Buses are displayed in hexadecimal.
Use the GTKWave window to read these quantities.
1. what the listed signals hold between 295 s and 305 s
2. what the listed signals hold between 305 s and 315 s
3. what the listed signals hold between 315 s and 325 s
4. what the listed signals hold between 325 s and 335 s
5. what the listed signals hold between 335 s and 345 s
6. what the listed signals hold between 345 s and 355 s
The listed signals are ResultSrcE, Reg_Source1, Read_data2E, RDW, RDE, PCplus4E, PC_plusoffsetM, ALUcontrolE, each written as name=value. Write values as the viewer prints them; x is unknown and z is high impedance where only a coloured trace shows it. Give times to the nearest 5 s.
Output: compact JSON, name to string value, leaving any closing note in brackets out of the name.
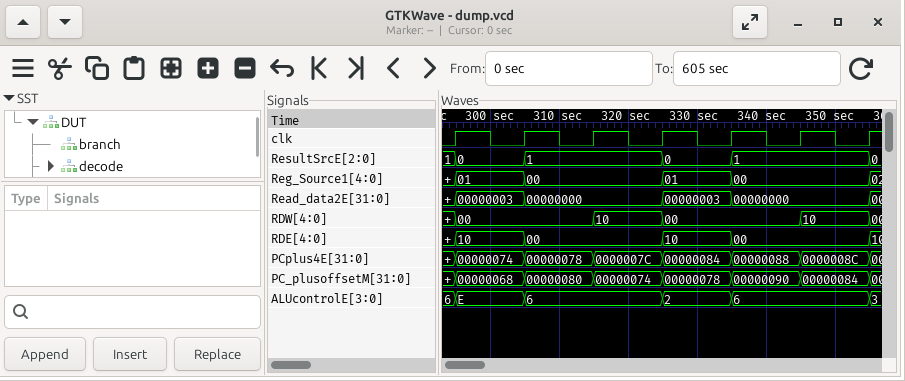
{"what the listed signals hold between 295 s and 305 s": "ResultSrcE=0, Reg_Source1=01, Read_data2E=00000003, RDW=00, RDE=10, PCplus4E=00000074, PC_plusoffsetM=00000068, ALUcontrolE=E", "what the listed signals hold between 305 s and 315 s": "ResultSrcE=1, Reg_Source1=00, Read_data2E=00000000, RDW=00, RDE=00, PCplus4E=00000078, PC_plusoffsetM=00000080, ALUcontrolE=6", "what the listed signals hold between 315 s and 325 s": "ResultSrcE=1, Reg_Source1=00, Read_data2E=00000000, RDW=10, RDE=00, PCplus4E=0000007C, PC_plusoffsetM=00000074, ALUcontrolE=6", "what the listed signals hold between 325 s and 335 s": "ResultSrcE=0, Reg_Source1=01, Read_data2E=00000003, RDW=00, RDE=10, PCplus4E=00000084, PC_plusoffsetM=00000078, ALUcontrolE=2", "what the listed signals hold between 335 s and 345 s": "ResultSrcE=1, Reg_Source1=00, Read_data2E=00000000, RDW=00, RDE=00, PCplus4E=00000088, PC_plusoffsetM=00000090, ALUcontrolE=6", "what the listed signals hold between 345 s and 355 s": "ResultSrcE=1, Reg_Source1=00, Read_data2E=00000000, RDW=10, RDE=00, PCplus4E=0000008C, PC_plusoffsetM=00000084, ALUcontrolE=6"}
